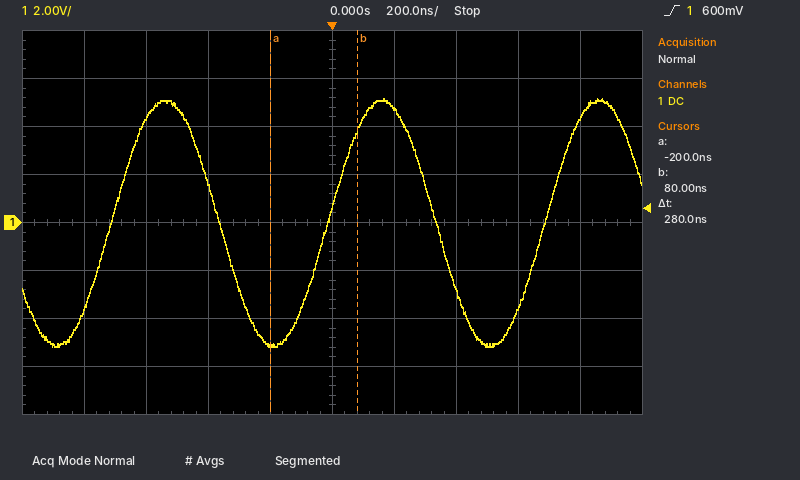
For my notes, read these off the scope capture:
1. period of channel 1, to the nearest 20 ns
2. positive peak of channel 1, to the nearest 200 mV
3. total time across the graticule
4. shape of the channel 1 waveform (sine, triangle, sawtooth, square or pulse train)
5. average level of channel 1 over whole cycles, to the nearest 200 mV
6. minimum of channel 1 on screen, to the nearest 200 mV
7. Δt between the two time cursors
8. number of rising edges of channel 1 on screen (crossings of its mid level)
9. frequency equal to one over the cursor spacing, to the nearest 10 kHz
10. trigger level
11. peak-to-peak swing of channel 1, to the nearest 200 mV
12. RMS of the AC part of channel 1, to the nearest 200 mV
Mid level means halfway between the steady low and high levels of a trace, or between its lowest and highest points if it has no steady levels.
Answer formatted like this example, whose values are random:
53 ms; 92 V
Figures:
700 ns; 5.2 V; 2 µs; sine; 0.0 V; -5.2 V; 280 ns; 3; 3.57 MHz; 600 mV; 10.4 V; 3.6 V
